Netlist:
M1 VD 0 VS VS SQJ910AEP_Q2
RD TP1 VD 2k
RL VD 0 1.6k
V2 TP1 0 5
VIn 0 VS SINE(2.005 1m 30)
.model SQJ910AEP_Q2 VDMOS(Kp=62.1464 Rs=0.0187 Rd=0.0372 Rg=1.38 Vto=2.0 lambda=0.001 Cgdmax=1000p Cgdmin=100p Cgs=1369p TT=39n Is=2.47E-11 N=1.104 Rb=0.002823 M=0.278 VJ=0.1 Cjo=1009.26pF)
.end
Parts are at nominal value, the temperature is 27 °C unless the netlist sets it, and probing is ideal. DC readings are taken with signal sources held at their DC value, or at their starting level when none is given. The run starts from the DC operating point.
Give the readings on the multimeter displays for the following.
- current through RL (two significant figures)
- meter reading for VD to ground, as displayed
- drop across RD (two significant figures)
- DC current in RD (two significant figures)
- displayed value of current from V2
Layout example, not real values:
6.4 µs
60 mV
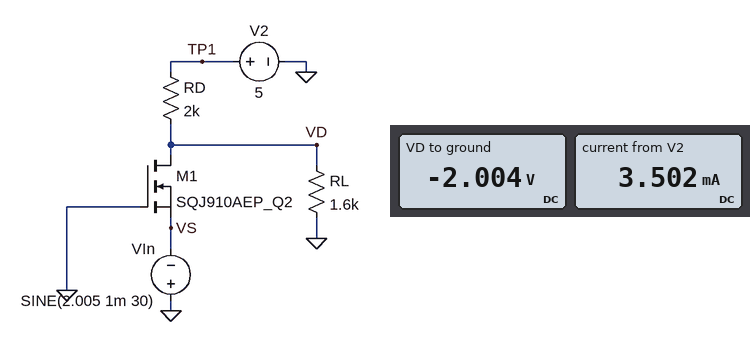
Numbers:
1.3 mA
-2.004 V
7.0 V
3.5 mA
3.502 mA
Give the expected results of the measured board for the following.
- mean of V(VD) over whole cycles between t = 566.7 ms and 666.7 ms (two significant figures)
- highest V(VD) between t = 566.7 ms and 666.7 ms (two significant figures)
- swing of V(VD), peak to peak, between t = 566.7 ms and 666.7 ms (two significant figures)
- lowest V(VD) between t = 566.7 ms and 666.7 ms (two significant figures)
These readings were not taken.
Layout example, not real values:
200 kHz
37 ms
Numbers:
-2.0 V
-2.0 V
2.0 mV
-2.0 V
